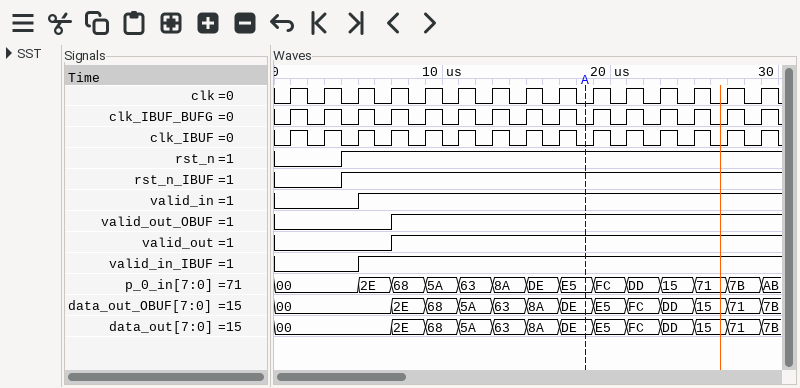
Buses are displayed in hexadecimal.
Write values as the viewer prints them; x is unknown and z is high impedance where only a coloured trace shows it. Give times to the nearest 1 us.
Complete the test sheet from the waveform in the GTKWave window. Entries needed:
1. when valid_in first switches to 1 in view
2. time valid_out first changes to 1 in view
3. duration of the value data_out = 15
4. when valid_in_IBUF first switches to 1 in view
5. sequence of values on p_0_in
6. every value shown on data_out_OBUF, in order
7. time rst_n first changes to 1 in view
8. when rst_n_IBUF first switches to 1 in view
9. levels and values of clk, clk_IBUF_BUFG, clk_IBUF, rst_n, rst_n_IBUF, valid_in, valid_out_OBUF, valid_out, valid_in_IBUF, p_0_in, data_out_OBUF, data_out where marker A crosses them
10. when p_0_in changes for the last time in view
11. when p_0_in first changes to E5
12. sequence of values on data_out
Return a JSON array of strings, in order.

["5 us", "7 us", "2 us", "5 us", "00, 2E, 68, 5A, 63, 8A, DE, E5, FC, DD, 15, 71, 7B, AB", "00, 2E, 68, 5A, 63, 8A, DE, E5, FC, DD, 15, 71, 7B", "4 us", "4 us", "clk=0, clk_IBUF_BUFG=0, clk_IBUF=0, rst_n=1, rst_n_IBUF=1, valid_in=1, valid_out_OBUF=1, valid_out=1, valid_in_IBUF=1, p_0_in=E5, data_out_OBUF=DE, data_out=DE", "29 us", "17 us", "00, 2E, 68, 5A, 63, 8A, DE, E5, FC, DD, 15, 71, 7B"]
